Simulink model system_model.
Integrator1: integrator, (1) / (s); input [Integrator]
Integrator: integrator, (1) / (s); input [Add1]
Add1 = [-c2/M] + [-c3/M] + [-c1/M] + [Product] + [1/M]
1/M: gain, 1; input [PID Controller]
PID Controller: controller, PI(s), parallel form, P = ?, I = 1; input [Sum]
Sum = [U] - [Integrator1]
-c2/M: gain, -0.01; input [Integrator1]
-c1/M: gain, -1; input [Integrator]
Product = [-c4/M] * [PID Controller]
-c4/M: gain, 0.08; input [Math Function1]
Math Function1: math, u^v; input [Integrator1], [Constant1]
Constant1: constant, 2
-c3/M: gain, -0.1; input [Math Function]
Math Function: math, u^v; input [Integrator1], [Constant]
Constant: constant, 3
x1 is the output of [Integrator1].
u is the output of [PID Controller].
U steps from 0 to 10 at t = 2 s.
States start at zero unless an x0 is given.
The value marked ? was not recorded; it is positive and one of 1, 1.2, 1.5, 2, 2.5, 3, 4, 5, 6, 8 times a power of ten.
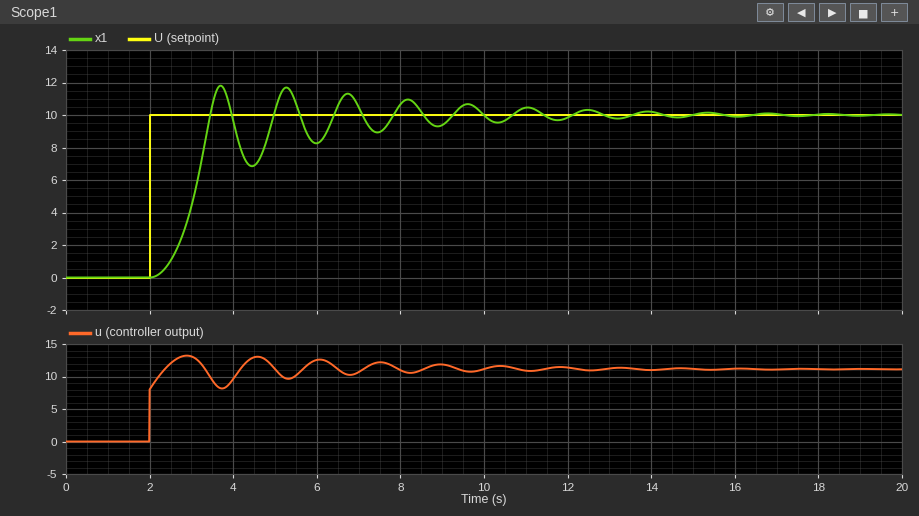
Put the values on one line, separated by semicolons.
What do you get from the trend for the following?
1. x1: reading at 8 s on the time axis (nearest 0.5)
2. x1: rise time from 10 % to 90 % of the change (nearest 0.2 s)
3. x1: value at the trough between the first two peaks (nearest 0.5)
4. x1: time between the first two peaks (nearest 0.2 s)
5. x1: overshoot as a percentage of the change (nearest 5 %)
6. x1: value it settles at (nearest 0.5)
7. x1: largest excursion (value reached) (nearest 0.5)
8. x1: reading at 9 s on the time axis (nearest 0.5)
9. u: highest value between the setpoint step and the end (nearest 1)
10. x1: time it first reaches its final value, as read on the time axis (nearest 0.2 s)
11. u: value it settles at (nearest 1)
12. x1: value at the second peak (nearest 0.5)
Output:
10.5; 0.8 s; 7.0; 1.6 s; 20 %; 10.0; 12.0; 9.5; 13; 3.4 s; 11; 11.5
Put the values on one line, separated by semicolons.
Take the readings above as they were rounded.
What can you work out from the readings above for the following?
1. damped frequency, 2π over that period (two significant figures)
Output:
3.9 rad/s
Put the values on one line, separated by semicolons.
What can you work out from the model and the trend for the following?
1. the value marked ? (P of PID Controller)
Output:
0.8
